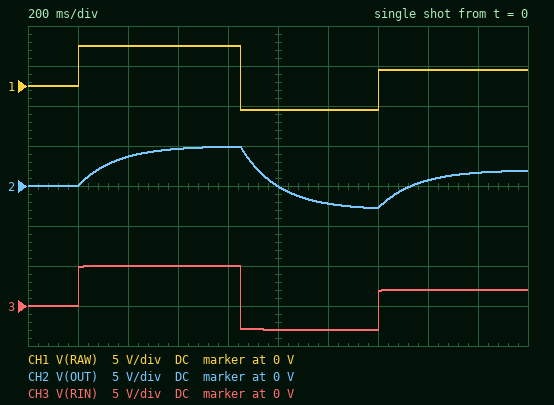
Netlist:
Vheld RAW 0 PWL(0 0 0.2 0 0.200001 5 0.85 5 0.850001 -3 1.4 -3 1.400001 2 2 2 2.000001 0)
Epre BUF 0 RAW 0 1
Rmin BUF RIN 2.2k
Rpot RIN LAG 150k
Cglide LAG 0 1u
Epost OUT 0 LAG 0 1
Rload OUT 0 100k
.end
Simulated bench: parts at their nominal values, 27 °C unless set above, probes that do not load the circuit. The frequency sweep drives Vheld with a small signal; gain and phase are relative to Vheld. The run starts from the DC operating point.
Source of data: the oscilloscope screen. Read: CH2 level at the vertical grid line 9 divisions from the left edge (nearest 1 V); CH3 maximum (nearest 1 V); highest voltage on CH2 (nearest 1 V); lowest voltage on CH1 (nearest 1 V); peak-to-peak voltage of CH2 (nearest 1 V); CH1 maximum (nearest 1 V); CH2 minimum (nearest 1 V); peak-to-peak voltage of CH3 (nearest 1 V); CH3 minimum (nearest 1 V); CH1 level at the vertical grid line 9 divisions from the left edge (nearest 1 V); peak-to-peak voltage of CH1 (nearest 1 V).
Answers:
2 V
5 V
5 V
-3 V
8 V
5 V
-3 V
8 V
-3 V
2 V
8 V
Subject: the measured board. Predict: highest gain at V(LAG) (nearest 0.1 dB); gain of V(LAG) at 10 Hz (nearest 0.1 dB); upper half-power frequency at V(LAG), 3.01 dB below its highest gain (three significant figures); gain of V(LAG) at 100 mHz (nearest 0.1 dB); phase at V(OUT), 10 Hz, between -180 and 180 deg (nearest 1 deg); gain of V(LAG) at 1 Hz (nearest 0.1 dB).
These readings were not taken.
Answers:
0 dB
-19.7 dB
1.05 Hz
0 dB
-84 deg
-2.8 dB
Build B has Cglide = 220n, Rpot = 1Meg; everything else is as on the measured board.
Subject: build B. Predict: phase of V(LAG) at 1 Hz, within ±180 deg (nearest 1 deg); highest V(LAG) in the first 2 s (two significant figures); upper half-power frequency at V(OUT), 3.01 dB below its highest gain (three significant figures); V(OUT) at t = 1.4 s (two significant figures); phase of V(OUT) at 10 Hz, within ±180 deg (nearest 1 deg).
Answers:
-54 deg
4.7 V
722 mHz
-2.4 V
-86 deg
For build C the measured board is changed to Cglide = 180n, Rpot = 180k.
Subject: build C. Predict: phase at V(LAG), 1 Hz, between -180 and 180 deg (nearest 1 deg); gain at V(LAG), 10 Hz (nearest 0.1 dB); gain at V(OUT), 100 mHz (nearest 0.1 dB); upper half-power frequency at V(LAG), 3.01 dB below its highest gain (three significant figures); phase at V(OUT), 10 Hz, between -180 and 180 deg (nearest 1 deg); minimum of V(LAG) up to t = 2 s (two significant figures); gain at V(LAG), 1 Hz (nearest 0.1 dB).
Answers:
-12 deg
-7.2 dB
0 dB
4.85 Hz
-64 deg
-3.0 V
-0.2 dB
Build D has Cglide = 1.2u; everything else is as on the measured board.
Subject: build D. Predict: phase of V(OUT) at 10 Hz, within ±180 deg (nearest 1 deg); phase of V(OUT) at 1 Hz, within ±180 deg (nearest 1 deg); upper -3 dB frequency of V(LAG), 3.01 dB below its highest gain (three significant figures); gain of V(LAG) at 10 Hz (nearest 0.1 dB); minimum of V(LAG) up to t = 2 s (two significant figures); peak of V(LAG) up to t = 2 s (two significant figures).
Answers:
-85 deg
-49 deg
871 mHz
-21.2 dB
-2.6 V
4.9 V
